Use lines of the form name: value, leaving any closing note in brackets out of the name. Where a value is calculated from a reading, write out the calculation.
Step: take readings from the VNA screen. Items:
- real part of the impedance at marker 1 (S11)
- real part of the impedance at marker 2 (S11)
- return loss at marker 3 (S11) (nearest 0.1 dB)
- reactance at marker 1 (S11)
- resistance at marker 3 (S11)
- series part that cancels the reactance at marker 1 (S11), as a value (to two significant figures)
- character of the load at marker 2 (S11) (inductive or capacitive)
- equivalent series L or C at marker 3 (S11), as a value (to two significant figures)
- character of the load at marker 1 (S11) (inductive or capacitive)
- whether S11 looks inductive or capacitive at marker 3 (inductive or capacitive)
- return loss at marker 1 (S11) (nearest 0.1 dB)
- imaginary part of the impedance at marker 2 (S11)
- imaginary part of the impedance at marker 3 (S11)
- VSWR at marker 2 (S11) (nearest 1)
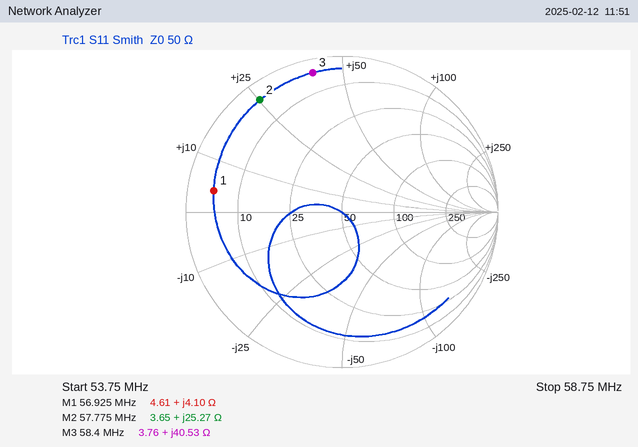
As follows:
real part of the impedance at marker 1: 4.61 Ω
real part of the impedance at marker 2: 3.65 Ω
return loss at marker 3 (S11): 0.8 dB
reactance at marker 1: +4.10 Ω
resistance at marker 3: 3.76 Ω
series part that cancels the reactance at marker 1 (S11), as a value: C = 1/(2π × 56.925 MHz × 4.1 Ω) ≈ 682 pF, so 680 pF to two significant figures
character of the load at marker 2 (S11): inductive
equivalent series L or C at marker 3 (S11), as a value: L = 40.53 Ω/(2π × 58.4 MHz) ≈ 110 nH
character of the load at marker 1 (S11): inductive
whether S11 looks inductive or capacitive at marker 3: inductive
return loss at marker 1 (S11): 1.6 dB
imaginary part of the impedance at marker 2: +25.27 Ω
imaginary part of the impedance at marker 3: +40.53 Ω
VSWR at marker 2 (S11): 17
